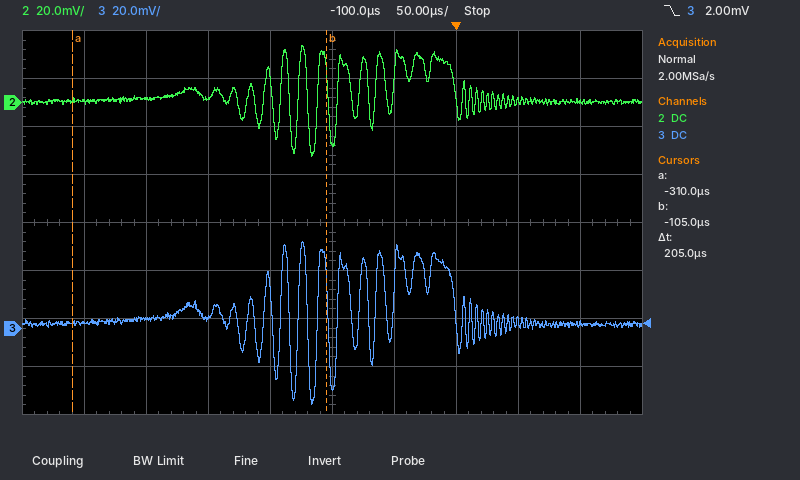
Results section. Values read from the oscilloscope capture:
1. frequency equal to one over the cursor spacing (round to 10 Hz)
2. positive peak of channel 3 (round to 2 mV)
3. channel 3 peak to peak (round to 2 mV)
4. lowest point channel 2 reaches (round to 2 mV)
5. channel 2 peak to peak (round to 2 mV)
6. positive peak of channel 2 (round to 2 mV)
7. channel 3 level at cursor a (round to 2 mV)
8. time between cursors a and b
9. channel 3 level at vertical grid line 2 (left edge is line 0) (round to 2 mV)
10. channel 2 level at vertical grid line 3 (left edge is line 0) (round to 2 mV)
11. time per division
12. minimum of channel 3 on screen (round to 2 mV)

4.88 kHz
36 mV
68 mV
-22 mV
46 mV
24 mV
2 mV
205 µs
4 mV
2 mV
50 µs
-32 mV
